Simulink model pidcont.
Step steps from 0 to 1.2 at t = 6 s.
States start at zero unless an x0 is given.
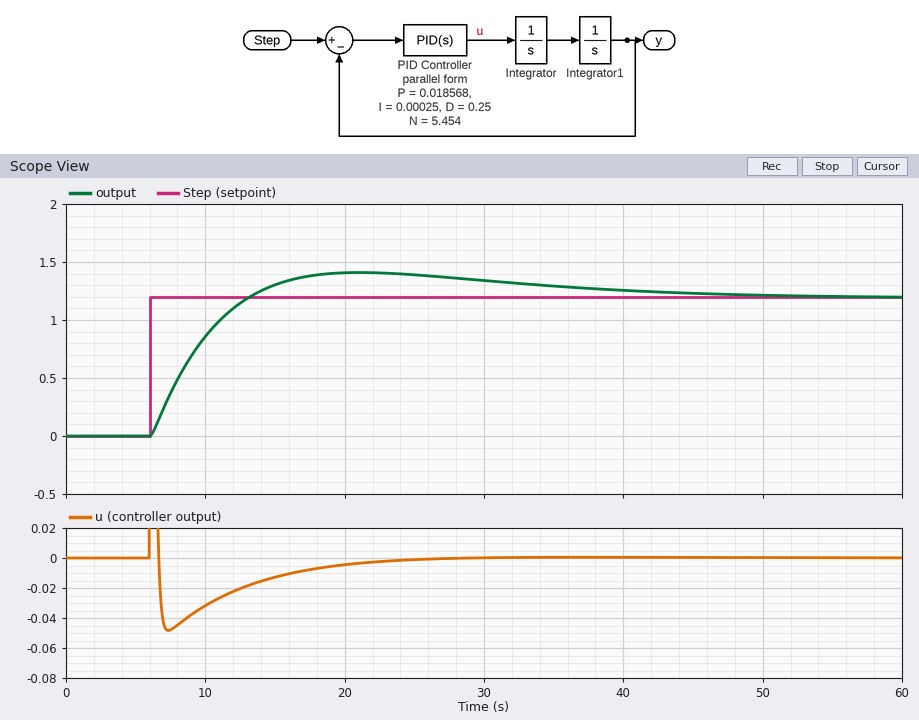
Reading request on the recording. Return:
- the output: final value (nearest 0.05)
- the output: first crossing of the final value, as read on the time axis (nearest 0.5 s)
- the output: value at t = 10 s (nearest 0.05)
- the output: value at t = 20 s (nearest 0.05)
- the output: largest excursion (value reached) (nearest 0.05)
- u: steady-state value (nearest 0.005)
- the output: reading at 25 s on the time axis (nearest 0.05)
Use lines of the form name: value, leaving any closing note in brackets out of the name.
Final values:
the output: final value: 1.20
the output: first crossing of the final value, as read on the time axis: 13.0 s
the output: value at t = 10 s: 0.85
the output: value at t = 20 s: 1.40
the output: largest excursion (value reached): 1.40
u: steady-state value: 0.000
the output: reading at 25 s on the time axis: 1.40
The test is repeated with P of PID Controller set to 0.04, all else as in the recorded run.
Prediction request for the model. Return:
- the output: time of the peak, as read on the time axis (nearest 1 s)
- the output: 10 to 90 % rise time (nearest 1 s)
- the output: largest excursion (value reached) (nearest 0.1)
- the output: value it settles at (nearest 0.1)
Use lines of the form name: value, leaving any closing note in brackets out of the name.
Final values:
the output: time of the peak, as read on the time axis: 17 s
the output: 10 to 90 % rise time: 4 s
the output: largest excursion (value reached): 1.5
the output: value it settles at: 1.2
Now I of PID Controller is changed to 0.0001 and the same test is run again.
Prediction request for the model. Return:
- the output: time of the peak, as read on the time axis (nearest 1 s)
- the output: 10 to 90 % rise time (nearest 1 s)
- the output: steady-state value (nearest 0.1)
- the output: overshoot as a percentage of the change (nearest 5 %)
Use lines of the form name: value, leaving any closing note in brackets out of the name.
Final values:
the output: time of the peak, as read on the time axis: 21 s
the output: 10 to 90 % rise time: 5 s
the output: steady-state value: 1.2
the output: overshoot as a percentage of the change: 15 %
